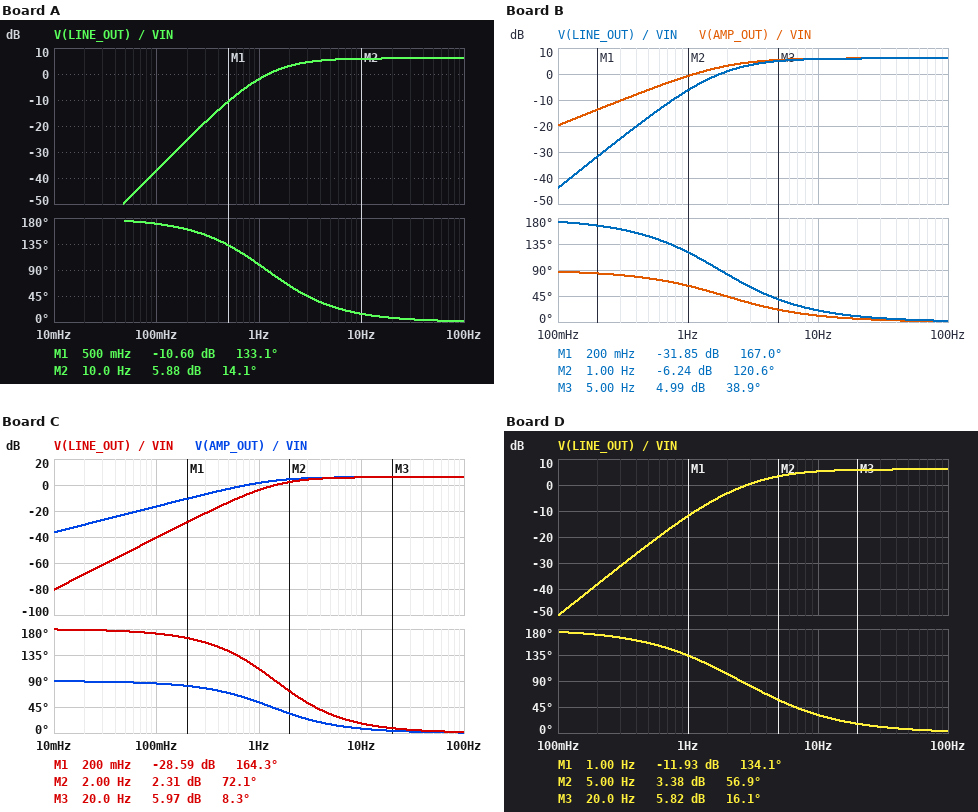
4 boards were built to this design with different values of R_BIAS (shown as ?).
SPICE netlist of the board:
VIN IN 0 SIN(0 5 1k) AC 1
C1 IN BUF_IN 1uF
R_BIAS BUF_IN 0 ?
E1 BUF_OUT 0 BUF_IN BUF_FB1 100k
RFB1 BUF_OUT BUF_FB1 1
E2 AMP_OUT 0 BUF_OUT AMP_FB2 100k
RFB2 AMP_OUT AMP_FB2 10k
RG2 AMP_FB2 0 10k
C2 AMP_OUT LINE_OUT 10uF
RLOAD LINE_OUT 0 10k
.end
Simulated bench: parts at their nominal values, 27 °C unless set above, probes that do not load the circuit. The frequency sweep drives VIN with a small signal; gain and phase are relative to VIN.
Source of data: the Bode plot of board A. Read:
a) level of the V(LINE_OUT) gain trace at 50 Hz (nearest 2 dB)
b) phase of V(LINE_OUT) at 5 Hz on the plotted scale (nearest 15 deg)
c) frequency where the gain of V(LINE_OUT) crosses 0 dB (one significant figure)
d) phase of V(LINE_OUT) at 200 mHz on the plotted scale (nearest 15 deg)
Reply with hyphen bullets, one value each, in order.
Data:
- 6 dB
- 30 deg
- 1 Hz
- 165 deg
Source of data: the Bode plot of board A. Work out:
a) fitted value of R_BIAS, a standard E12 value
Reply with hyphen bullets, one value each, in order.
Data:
- 180 kΩ
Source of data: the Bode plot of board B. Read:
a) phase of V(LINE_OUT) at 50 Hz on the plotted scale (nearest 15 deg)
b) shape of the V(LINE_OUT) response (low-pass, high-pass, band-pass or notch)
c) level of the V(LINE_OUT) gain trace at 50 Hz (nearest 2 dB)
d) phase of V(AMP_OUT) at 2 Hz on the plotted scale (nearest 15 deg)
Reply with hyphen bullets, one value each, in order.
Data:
- 0 deg
- high-pass
- 6 dB
- 45 deg
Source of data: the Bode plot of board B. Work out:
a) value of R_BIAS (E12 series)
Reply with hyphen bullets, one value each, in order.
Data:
- 82 kΩ
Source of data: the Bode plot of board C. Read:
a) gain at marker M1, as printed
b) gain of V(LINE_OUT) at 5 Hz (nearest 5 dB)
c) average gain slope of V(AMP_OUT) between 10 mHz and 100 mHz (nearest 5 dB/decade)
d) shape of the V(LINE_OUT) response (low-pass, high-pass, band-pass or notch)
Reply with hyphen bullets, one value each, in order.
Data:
- -28.59 dB
- 5 dB
- 20 dB/decade
- high-pass
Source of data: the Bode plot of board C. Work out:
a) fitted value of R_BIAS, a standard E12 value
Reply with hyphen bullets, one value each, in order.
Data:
- 120 kΩ
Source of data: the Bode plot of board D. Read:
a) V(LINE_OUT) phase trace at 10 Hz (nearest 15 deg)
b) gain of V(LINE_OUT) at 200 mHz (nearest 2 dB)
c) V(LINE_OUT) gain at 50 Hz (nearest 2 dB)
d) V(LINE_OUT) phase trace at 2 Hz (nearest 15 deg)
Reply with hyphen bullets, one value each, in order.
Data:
- 30 deg
- -38 dB
- 6 dB
- 105 deg
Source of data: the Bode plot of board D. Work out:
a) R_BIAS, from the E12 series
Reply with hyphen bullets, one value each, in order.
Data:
- 39 kΩ
